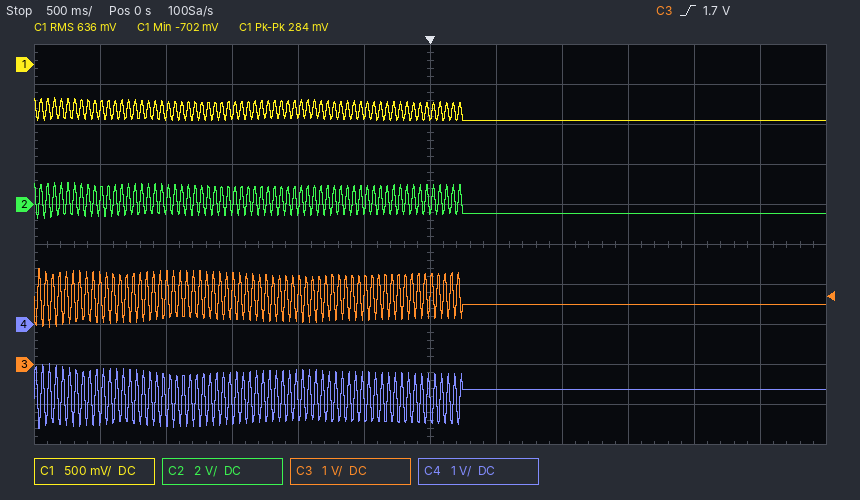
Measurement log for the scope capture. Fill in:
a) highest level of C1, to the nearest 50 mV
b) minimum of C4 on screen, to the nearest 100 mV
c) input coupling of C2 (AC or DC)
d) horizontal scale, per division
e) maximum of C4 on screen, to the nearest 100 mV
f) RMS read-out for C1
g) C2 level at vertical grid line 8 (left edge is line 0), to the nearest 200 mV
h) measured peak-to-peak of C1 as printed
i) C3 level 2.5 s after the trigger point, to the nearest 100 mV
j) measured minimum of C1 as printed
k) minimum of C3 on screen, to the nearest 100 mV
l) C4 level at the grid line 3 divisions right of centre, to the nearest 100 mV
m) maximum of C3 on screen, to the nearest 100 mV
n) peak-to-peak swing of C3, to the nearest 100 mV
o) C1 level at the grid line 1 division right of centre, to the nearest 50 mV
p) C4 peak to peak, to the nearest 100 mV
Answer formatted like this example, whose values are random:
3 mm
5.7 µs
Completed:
-400 mV
-2.6 V
DC
500 ms
-1.0 V
636 mV
-400 mV
284 mV
1.5 V
-702 mV
900 mV
-1.6 V
2.4 V
1.5 V
-700 mV
1.6 V
